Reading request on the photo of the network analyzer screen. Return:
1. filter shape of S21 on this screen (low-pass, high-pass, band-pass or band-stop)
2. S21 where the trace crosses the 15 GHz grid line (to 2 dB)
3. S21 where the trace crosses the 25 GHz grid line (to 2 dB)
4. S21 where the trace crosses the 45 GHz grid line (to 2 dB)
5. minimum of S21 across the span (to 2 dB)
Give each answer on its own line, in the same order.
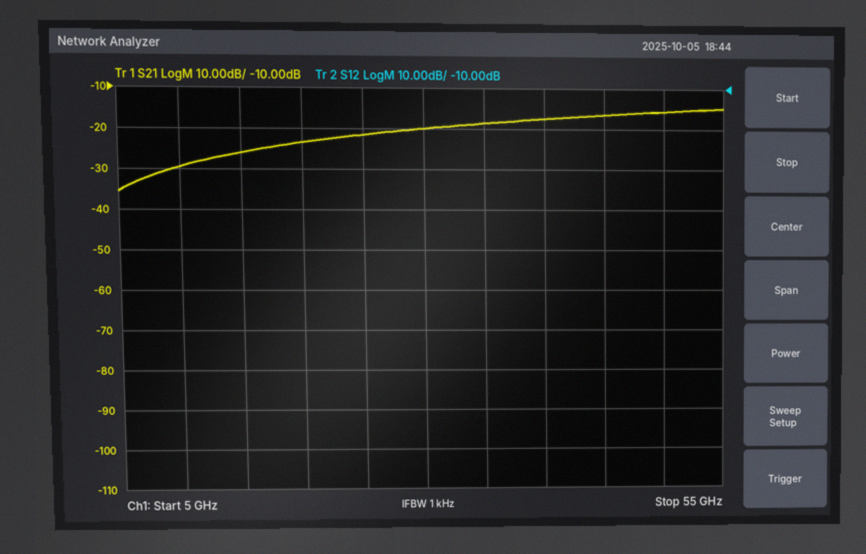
high-pass
-26 dB
-22 dB
-16 dB
-36 dB
